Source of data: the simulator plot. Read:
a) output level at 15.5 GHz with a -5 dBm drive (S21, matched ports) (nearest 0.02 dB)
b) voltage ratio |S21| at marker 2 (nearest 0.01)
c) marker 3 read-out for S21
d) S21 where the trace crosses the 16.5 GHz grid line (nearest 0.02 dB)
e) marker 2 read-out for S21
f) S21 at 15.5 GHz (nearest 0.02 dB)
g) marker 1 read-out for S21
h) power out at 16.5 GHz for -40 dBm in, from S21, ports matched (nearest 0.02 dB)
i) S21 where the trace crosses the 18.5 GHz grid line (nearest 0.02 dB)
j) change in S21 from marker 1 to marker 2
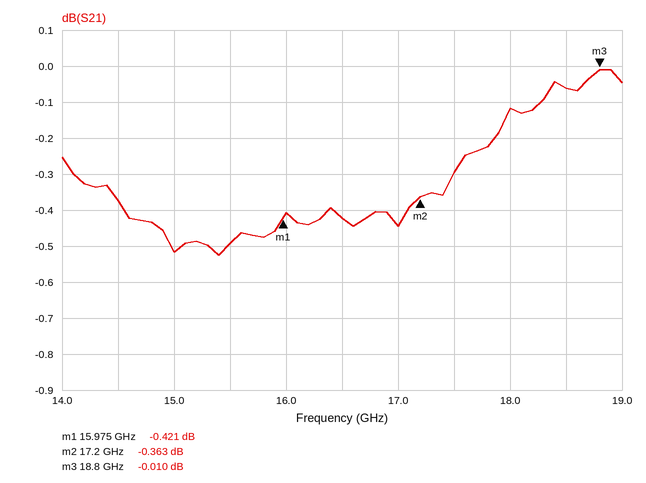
-5.50 dBm
0.96
-0.010 dB
-0.42 dB
-0.363 dB
-0.50 dB
-0.421 dB
-40.42 dBm
-0.06 dB
0.058 dB
